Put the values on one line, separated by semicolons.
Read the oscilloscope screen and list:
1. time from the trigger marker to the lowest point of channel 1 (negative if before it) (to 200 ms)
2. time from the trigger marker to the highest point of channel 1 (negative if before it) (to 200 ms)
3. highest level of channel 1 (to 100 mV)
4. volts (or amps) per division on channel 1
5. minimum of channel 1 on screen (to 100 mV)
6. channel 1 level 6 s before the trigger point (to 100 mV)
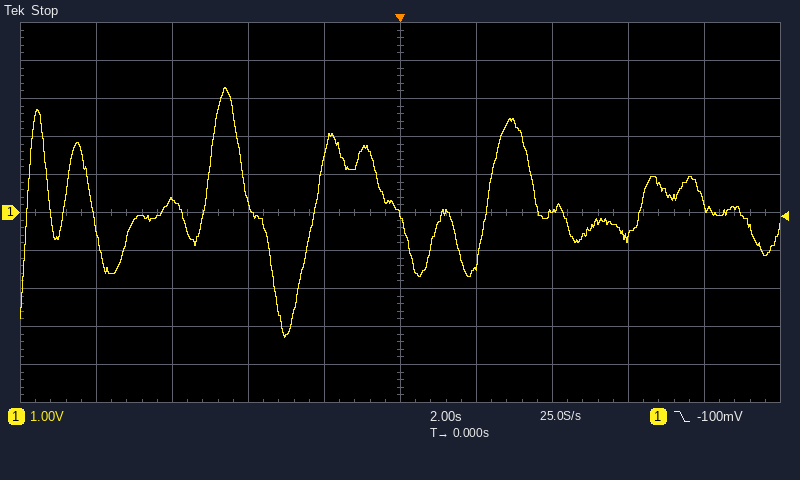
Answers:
-3.0 s; -4.6 s; 3.3 V; 1 V; -3.3 V; 300 mV
